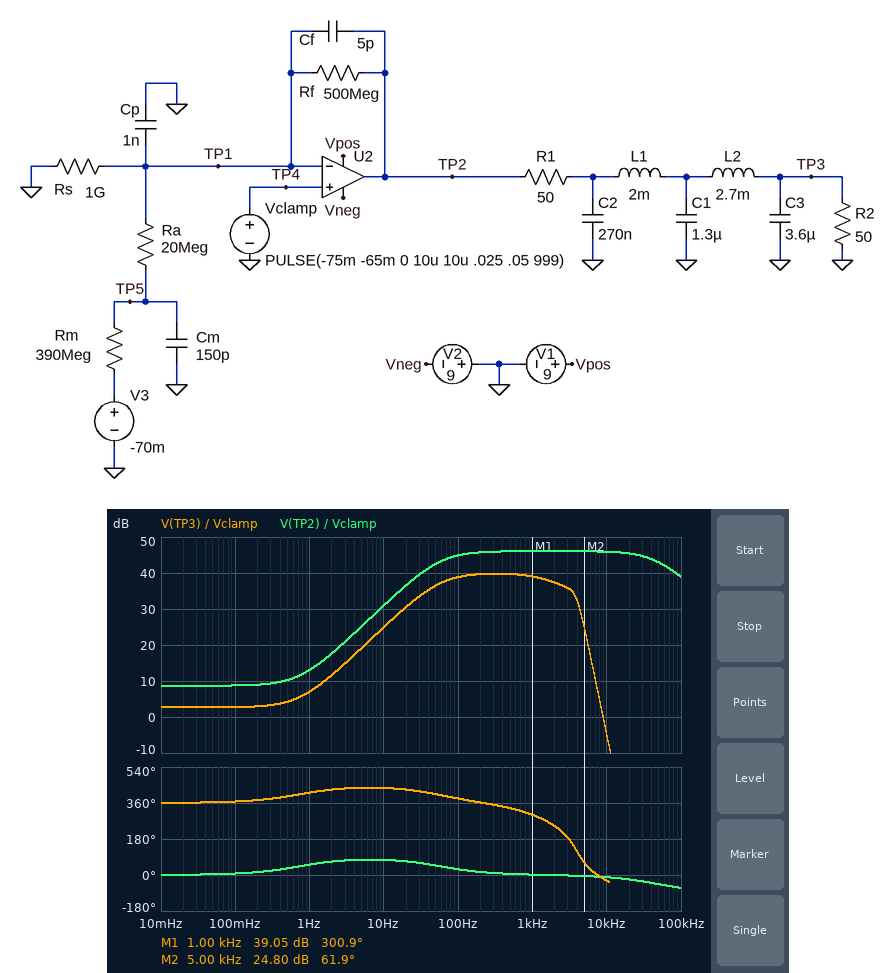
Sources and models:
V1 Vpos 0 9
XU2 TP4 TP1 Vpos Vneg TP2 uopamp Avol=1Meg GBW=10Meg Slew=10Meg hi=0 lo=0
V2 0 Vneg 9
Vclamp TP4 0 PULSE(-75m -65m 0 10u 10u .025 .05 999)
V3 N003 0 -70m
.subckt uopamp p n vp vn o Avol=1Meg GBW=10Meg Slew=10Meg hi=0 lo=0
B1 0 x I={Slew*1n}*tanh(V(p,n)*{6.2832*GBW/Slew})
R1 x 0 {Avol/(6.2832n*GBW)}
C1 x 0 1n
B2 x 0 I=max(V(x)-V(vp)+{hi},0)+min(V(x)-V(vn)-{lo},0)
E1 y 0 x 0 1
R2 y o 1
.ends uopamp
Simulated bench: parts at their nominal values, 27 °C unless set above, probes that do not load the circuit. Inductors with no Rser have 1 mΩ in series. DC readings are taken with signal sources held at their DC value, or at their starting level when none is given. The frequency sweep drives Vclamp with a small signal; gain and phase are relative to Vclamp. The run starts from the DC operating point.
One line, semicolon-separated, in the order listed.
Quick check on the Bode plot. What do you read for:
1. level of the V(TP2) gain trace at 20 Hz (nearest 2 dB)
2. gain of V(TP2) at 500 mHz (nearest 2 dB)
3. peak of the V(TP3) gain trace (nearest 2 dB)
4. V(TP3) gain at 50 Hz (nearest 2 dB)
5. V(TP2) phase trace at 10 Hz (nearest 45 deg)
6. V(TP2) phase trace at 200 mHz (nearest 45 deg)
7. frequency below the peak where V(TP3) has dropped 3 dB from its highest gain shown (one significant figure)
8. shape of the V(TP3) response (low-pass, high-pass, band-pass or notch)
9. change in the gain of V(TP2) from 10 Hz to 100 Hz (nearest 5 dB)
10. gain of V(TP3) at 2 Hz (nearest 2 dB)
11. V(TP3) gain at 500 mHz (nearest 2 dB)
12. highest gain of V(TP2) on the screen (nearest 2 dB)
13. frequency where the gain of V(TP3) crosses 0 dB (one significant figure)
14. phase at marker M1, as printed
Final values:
36 dB; 10 dB; 40 dB; 36 dB; 90 deg; 0 deg; 50 Hz; band-pass; 15 dB; 12 dB; 4 dB; 46 dB; 9 kHz; 300.9 deg
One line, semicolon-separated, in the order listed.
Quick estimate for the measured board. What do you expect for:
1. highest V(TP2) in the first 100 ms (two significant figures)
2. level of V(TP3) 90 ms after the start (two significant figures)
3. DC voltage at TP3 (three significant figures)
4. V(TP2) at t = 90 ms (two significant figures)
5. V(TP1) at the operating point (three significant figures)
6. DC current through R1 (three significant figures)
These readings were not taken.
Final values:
1.9 V; -65 mV; -59.3 mV; -130 mV; -75.0 mV; 1.19 mA
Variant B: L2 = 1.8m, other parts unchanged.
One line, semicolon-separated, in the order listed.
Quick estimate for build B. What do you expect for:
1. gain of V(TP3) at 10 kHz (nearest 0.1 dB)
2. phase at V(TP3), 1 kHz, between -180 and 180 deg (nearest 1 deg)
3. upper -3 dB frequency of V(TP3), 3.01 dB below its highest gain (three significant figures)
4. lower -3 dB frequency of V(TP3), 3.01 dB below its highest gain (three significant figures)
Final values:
-0.8 dB; -55 deg; 2.04 kHz; 52.8 Hz
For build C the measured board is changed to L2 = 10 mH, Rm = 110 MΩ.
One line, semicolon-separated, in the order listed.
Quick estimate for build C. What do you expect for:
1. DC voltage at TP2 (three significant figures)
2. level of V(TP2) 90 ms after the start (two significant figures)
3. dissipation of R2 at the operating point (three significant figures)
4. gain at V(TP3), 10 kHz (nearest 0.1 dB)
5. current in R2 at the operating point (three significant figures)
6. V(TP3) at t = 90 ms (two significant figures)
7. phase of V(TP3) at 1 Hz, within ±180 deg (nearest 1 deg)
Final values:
-132 mV; -140 mV; 86.8 µW; -16.9 dB; 1.32 mA; -70 mV; 32 deg
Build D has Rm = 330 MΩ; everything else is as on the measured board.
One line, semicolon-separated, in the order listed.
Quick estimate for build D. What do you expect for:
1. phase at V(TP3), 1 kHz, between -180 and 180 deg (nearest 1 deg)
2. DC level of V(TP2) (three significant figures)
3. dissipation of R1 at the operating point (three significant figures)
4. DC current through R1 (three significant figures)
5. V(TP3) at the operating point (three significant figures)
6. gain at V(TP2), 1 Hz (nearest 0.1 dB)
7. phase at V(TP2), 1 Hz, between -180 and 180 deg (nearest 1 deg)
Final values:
-59 deg; -120 mV; 71.6 µW; 1.20 mA; -59.8 mV; 13.3 dB; 50 deg
